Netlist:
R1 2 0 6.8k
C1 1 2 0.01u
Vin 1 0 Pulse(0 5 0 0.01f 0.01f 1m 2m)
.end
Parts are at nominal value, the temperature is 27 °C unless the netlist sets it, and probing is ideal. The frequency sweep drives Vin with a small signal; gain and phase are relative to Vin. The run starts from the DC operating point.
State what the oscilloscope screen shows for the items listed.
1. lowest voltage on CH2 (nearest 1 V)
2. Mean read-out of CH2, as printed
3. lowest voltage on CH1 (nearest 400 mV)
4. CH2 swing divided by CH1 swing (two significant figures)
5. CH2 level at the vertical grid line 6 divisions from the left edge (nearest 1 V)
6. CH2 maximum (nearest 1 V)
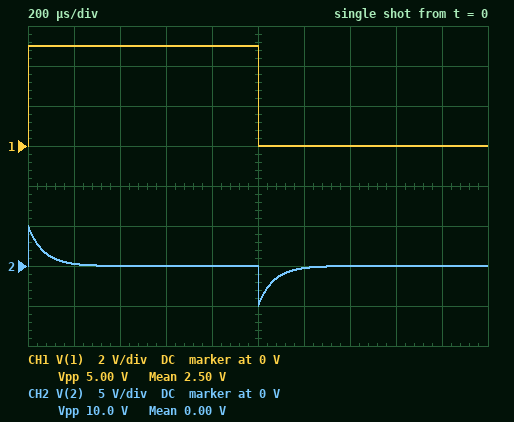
-5 V
0.00 V
0 V
2.0
0 V
5 V
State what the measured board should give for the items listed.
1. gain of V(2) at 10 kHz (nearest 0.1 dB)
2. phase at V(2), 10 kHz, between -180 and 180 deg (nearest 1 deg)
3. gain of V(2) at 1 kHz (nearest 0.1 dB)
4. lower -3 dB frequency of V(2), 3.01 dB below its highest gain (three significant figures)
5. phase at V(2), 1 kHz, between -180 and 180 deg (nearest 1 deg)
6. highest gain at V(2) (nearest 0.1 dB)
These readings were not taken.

-0.2 dB
13 deg
-8.1 dB
2.34 kHz
67 deg
0 dB
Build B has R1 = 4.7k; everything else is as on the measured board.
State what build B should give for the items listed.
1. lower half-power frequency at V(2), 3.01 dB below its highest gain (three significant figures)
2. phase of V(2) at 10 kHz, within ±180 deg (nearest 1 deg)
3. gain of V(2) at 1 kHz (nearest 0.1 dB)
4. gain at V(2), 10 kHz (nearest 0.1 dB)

3.39 kHz
19 deg
-11.0 dB
-0.5 dB
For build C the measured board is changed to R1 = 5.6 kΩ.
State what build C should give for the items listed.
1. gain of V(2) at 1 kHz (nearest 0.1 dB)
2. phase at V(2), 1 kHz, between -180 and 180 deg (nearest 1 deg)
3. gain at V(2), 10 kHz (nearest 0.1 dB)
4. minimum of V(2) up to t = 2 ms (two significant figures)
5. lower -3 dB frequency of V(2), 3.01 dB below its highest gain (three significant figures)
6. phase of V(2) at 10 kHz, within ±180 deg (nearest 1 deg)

-9.6 dB
71 deg
-0.3 dB
-5.0 V
2.84 kHz
16 deg
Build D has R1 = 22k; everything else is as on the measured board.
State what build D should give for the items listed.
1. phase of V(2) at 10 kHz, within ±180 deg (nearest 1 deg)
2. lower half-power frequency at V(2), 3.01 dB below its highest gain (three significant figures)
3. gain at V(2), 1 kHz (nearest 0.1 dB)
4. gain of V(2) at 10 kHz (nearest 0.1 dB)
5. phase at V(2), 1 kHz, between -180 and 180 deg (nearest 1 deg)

4 deg
723 Hz
-1.8 dB
0 dB
36 deg
